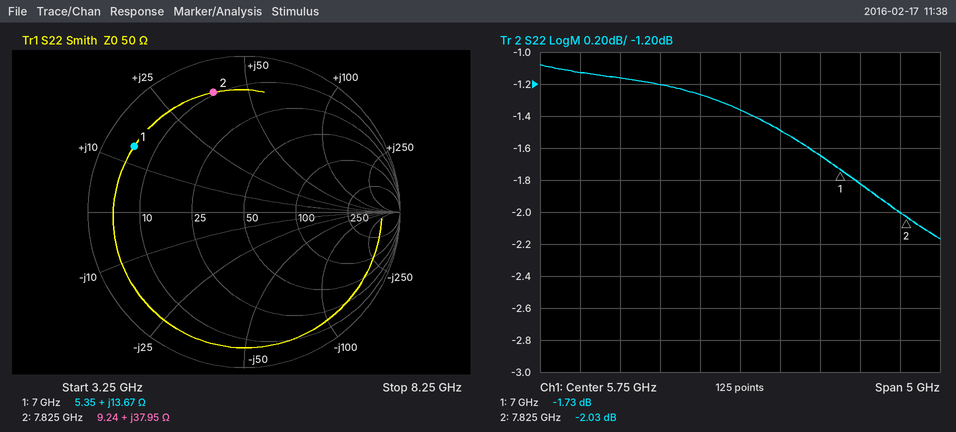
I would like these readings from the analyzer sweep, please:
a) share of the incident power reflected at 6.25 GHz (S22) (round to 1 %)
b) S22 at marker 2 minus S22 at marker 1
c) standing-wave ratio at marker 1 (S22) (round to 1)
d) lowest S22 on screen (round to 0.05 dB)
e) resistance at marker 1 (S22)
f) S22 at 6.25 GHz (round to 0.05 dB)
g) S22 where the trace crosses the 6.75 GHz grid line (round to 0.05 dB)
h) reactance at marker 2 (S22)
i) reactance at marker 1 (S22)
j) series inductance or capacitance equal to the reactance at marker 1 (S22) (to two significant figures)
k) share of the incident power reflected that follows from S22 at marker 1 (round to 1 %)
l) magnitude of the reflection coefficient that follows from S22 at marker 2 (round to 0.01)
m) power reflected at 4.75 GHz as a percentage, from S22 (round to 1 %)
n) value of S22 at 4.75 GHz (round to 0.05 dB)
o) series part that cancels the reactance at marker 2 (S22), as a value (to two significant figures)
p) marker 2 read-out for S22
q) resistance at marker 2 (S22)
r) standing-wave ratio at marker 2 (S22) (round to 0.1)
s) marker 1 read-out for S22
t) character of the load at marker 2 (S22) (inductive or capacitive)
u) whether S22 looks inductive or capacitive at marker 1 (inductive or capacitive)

71 %
-0.30 dB
10
-2.15 dB
5.35 Ω
-1.50 dB
-1.65 dB
+37.95 Ω
+13.67 Ω
310 pH
67 %
0.79
76 %
-1.20 dB
540 fF
-2.03 dB
9.24 Ω
8.6
-1.73 dB
inductive
inductive
